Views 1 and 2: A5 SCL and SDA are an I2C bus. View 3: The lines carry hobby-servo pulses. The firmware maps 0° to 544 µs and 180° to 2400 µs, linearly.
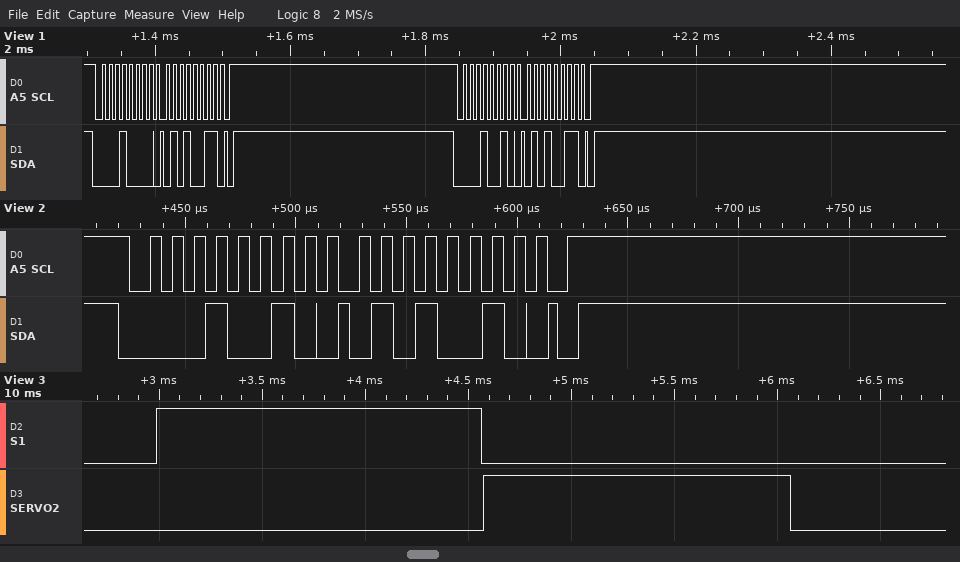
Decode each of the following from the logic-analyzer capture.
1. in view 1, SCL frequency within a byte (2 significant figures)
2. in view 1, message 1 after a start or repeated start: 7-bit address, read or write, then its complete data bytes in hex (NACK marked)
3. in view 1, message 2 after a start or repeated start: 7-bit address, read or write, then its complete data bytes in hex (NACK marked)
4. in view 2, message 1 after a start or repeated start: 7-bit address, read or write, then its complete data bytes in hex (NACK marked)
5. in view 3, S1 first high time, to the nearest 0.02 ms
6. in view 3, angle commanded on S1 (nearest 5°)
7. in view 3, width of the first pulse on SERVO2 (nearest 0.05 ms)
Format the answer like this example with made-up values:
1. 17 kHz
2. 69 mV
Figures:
1. 100 kHz
2. 0x08 write: 53
3. 0x09 write: 53
4. 0x09 write: 52
5. 1.58 ms
6. 100°
7. 1.50 ms
